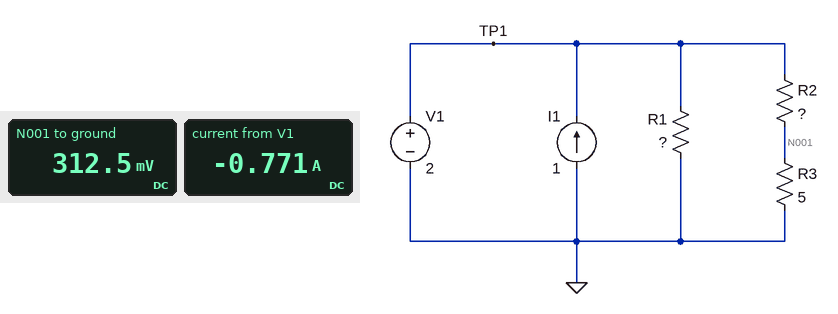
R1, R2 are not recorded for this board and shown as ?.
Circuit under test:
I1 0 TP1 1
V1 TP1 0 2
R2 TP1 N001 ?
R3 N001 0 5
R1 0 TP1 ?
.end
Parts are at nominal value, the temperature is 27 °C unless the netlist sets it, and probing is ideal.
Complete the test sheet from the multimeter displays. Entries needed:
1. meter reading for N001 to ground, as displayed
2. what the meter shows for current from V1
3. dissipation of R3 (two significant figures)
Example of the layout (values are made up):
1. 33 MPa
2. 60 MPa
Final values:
1. 312.5 mV
2. -0.771 A
3. 20 mW
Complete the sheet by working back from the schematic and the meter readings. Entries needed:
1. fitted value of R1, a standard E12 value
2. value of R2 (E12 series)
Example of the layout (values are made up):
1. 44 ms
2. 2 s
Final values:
1. 12 Ω
2. 27 Ω
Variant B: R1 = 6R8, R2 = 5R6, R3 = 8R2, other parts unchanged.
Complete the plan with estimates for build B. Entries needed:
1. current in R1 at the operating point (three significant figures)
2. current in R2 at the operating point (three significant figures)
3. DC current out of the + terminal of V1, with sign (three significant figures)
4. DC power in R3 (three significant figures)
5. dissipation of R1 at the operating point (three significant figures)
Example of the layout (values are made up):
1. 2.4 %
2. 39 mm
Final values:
1. 294 mA
2. 145 mA
3. -561 mA
4. 172 mW
5. 588 mW
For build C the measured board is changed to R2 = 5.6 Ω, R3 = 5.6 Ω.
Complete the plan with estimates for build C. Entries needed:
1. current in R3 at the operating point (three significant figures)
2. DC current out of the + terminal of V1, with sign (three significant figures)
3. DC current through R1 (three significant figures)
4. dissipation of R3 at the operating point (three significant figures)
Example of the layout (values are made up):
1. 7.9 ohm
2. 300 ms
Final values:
1. 179 mA
2. -655 mA
3. 167 mA
4. 179 mW
